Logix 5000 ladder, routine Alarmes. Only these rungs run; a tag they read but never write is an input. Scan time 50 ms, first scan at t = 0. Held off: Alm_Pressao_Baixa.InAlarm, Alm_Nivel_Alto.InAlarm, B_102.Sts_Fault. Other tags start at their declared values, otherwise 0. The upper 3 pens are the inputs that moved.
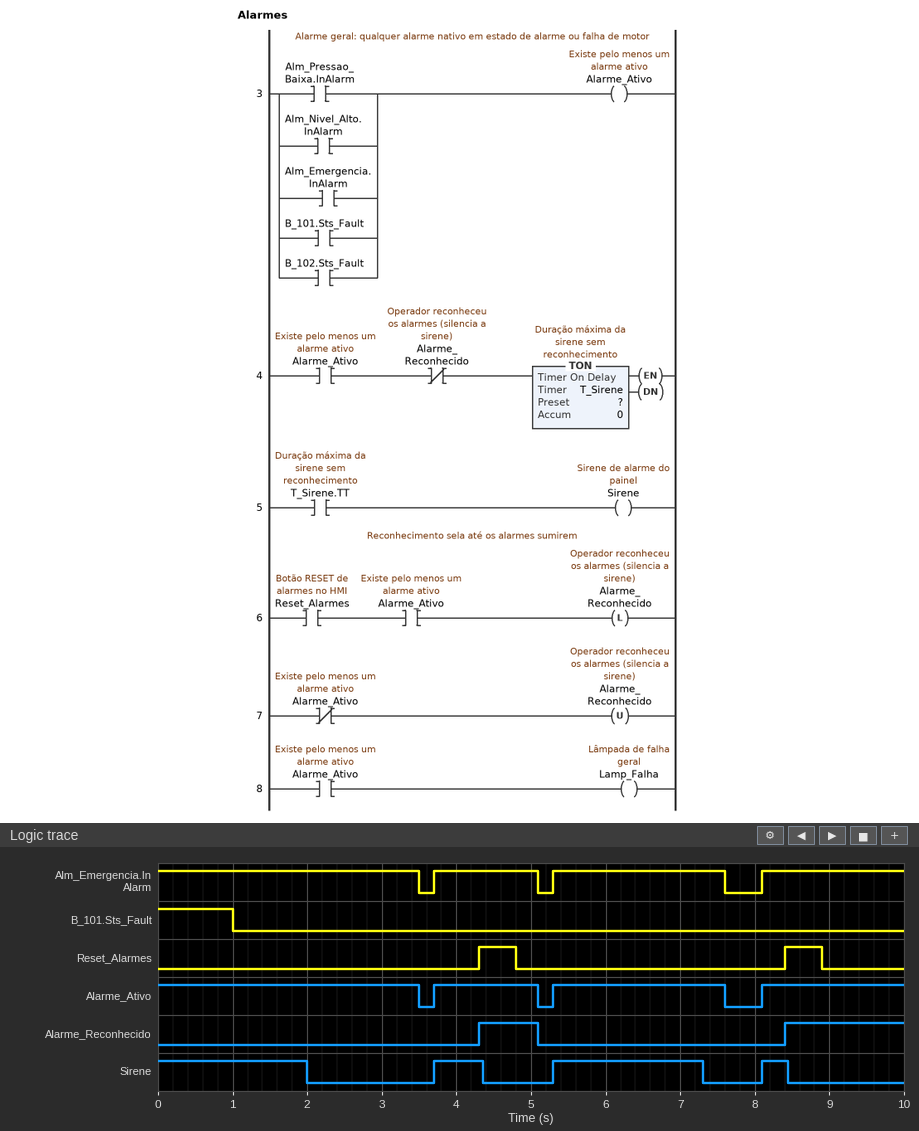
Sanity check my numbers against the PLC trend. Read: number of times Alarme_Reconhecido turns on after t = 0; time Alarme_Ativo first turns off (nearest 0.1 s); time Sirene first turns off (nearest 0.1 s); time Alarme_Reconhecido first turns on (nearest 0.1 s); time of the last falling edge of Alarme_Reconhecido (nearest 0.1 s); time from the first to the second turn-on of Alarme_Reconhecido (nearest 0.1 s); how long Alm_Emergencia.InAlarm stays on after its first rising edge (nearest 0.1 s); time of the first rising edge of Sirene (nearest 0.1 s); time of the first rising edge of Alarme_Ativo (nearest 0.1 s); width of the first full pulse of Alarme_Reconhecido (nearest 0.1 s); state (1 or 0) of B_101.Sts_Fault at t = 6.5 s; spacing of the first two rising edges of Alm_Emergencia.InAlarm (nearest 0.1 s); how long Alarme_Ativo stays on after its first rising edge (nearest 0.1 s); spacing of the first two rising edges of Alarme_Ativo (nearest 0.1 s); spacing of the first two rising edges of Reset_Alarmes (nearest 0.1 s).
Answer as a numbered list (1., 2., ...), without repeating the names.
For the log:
1. 2
2. 3.5 s
3. 2.0 s
4. 4.3 s
5. 5.1 s
6. 4.1 s
7. 1.4 s
8. 3.7 s
9. 3.7 s
10. 0.8 s
11. 0
12. 1.6 s
13. 1.4 s
14. 1.6 s
15. 4.1 s
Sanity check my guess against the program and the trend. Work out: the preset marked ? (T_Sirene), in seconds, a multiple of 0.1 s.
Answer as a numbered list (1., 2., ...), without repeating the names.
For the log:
1. 2.0 s
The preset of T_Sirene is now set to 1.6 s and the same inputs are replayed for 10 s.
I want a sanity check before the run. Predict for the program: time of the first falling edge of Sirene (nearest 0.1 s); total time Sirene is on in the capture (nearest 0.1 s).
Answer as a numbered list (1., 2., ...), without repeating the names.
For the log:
1. 1.6 s
2. 4.2 s
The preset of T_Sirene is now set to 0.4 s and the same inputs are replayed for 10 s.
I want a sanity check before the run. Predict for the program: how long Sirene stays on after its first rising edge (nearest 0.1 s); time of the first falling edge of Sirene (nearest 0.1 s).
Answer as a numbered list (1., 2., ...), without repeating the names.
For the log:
1. 0.4 s
2. 0.4 s
